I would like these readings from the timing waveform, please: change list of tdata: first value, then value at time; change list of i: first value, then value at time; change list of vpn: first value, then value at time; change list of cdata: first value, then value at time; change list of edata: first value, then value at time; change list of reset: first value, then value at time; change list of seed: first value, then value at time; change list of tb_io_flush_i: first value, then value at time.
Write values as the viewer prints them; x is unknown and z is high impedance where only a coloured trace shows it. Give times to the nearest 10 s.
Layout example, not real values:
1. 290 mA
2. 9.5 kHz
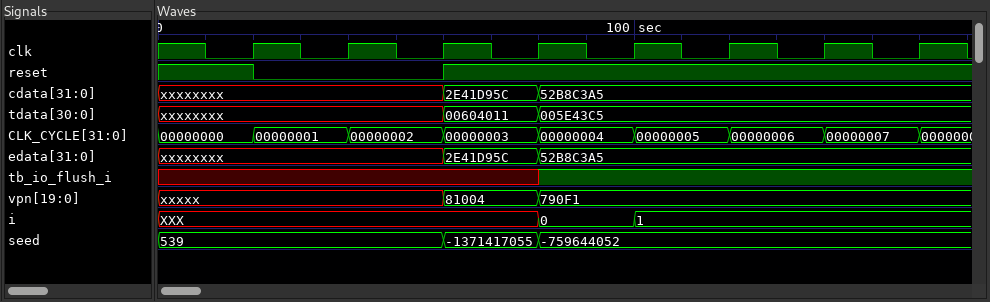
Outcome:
1. xxxxxxxx, 00604011 at 60 s, 005E43C5 at 80 s
2. XXX, 0 at 80 s, 1 at 100 s
3. xxxxx, 81004 at 60 s, 790F1 at 80 s
4. xxxxxxxx, 2E41D95C at 60 s, 52B8C3A5 at 80 s
5. xxxxxxxx, 2E41D95C at 60 s, 52B8C3A5 at 80 s
6. 1, 0 at 20 s, 1 at 60 s
7. 539, -1371417055 at 60 s, -759644052 at 80 s
8. x, 1 at 80 s
